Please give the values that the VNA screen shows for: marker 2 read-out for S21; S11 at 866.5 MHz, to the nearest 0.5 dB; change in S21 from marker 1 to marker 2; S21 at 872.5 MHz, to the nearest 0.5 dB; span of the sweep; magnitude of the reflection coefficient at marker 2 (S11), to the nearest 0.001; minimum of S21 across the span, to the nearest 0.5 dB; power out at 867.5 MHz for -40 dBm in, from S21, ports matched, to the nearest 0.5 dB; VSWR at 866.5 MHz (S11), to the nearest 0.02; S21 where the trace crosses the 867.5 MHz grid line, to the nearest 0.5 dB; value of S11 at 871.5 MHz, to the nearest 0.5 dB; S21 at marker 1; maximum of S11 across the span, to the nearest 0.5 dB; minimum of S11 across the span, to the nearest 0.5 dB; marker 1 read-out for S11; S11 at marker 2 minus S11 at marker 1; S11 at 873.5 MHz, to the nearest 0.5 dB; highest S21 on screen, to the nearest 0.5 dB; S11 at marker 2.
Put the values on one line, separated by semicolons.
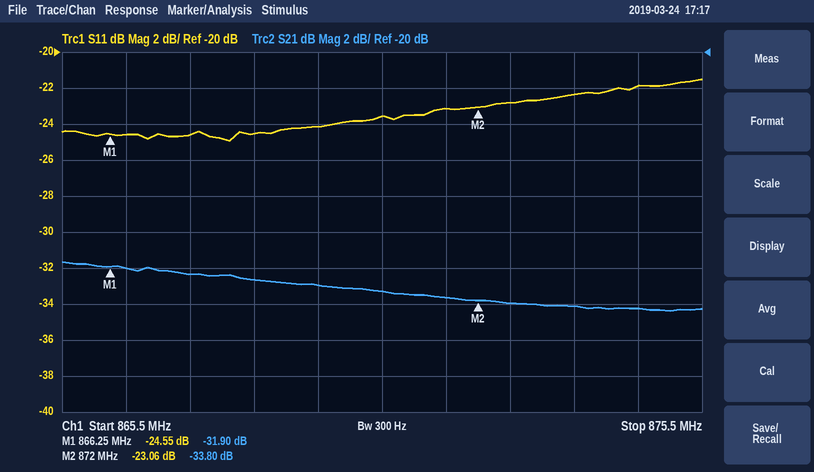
-33.80 dB; -24.5 dB; -1.90 dB; -34.0 dB; 10 MHz; 0.070; -34.5 dB; -72.5 dBm; 1.12; -32.5 dB; -23.0 dB; -31.90 dB; -21.5 dB; -25.0 dB; -24.55 dB; 1.49 dB; -22.5 dB; -31.5 dB; -23.06 dB
